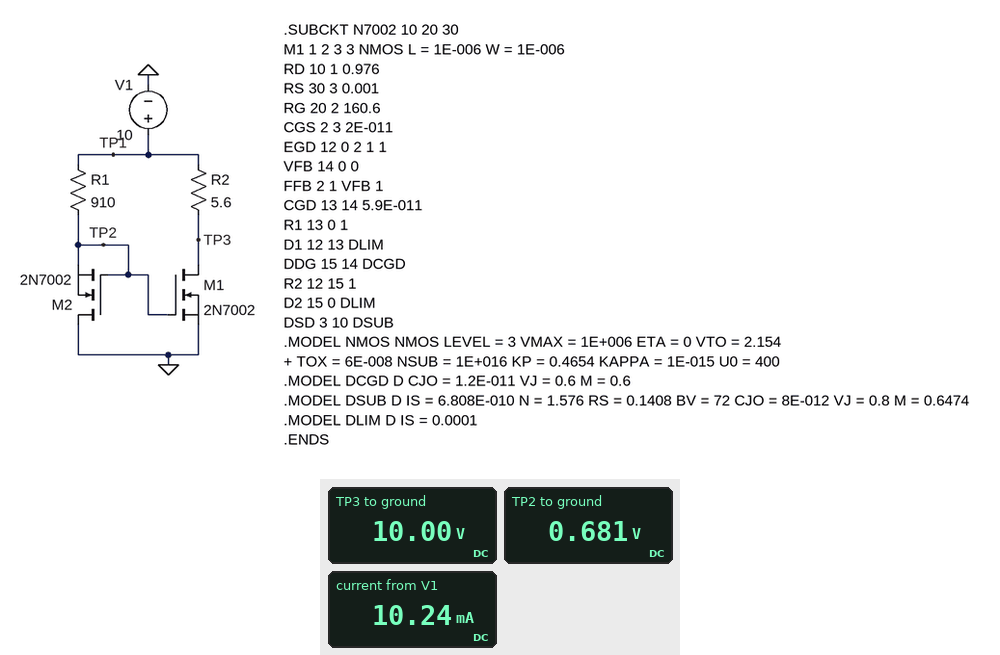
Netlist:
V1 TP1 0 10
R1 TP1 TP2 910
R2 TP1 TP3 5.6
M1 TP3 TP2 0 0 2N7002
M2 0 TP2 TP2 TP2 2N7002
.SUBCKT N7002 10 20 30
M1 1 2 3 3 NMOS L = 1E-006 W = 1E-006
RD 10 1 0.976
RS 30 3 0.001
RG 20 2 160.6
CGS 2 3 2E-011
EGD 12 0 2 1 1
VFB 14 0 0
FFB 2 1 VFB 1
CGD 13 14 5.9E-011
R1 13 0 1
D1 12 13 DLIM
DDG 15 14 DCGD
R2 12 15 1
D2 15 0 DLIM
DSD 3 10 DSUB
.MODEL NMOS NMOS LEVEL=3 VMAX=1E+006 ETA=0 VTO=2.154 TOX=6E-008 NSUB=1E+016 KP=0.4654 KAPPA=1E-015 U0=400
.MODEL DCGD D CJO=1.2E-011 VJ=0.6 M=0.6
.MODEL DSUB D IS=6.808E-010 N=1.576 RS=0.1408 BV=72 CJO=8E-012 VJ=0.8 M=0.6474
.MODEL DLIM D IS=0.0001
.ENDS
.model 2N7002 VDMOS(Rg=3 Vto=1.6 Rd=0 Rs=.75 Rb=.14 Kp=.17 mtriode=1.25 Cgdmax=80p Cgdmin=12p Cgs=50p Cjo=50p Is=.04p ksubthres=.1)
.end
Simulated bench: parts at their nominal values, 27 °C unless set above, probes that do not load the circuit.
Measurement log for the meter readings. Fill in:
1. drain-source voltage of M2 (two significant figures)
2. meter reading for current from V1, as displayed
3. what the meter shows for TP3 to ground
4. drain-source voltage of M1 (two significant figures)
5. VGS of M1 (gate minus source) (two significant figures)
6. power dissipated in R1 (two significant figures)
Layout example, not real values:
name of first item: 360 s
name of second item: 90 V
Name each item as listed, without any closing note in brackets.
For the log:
drain-source voltage of M2: -680 mV
meter reading for current from V1, as displayed: 10.24 mA
what the meter shows for TP3 to ground: 10.00 V
drain-source voltage of M1: 10 V
VGS of M1 (gate minus source): 680 mV
power dissipated in R1: 95 mW
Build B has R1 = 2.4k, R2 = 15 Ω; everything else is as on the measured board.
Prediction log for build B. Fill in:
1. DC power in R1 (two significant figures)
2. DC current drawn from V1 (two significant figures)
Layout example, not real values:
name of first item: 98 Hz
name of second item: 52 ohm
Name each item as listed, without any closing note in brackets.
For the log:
DC power in R1: 36 mW
DC current drawn from V1: 3.9 mA
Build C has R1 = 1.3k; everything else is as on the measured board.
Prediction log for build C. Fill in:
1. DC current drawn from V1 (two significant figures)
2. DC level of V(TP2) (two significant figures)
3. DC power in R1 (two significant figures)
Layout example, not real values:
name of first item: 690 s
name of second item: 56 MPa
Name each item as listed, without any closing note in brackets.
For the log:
DC current drawn from V1: 7.2 mA
DC level of V(TP2): 670 mV
DC power in R1: 67 mW
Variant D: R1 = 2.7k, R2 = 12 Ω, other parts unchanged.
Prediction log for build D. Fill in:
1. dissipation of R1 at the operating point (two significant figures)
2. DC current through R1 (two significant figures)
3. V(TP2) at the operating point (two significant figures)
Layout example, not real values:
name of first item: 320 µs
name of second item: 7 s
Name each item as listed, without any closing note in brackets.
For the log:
dissipation of R1 at the operating point: 32 mW
DC current through R1: 3.5 mA
V(TP2) at the operating point: 650 mV
